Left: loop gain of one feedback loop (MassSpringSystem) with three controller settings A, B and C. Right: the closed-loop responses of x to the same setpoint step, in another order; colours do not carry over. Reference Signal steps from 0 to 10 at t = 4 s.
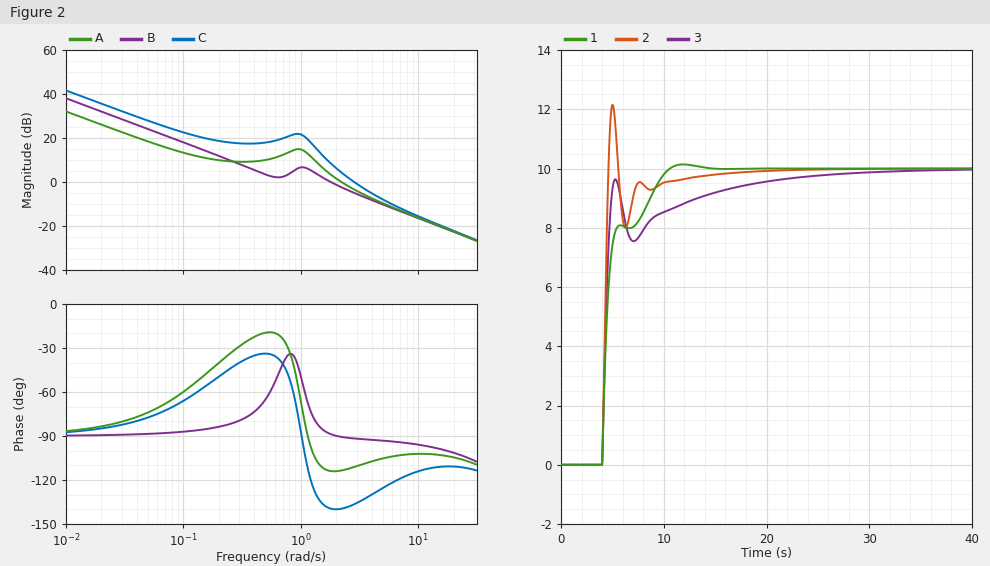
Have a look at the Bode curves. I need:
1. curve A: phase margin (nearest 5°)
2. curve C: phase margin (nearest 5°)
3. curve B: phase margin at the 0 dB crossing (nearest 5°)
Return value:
65°
45°
90°
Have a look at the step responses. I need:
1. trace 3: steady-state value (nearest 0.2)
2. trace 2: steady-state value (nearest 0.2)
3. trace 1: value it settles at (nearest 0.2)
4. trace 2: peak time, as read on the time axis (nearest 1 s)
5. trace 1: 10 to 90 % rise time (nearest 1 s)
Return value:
10.0
10.0
10.0
5 s
5 s
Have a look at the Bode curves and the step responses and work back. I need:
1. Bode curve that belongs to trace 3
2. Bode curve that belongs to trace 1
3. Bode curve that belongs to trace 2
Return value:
A
B
C
